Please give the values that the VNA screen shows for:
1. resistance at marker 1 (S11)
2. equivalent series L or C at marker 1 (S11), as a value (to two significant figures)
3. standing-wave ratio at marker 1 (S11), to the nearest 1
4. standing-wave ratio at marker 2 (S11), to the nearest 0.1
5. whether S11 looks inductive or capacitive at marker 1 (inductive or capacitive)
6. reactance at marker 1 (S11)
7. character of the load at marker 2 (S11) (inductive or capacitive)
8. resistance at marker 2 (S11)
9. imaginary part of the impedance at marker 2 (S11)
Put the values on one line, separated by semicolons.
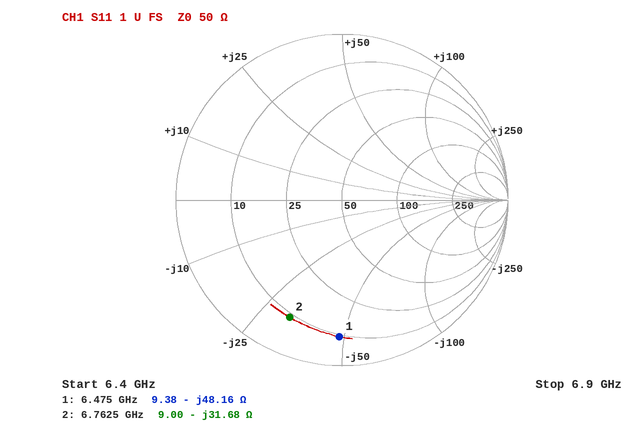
9.38 Ω; 510 fF; 10; 7.8; capacitive; -48.16 Ω; capacitive; 9.00 Ω; -31.68 Ω
